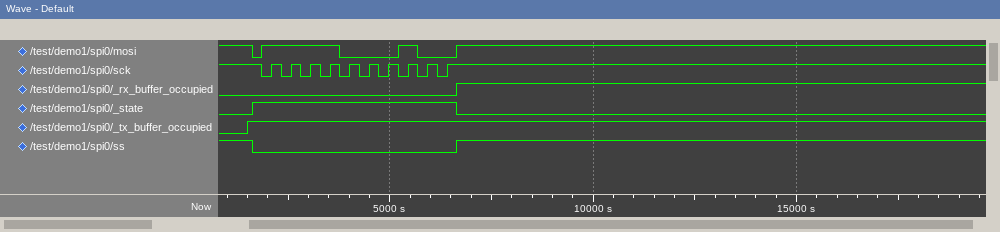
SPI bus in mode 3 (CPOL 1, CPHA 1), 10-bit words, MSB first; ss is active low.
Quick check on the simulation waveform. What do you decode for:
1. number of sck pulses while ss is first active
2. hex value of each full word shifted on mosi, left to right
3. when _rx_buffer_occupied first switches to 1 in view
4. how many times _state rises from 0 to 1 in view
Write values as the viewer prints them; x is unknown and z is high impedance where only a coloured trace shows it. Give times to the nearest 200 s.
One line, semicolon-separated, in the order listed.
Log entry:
10; 3C4; 6600 s; 1
